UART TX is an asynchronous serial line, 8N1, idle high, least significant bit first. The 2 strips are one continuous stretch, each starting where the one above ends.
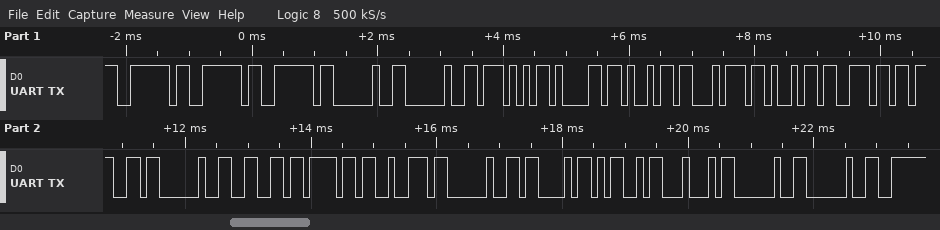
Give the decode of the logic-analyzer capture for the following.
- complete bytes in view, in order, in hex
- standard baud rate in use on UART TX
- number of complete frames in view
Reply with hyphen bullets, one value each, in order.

- 7E 7E 7E 20 20 57 61 69 74 69 6E 67 20 66 6F 72 20 43 4D 44 20 20
- 9600 baud
- 22
